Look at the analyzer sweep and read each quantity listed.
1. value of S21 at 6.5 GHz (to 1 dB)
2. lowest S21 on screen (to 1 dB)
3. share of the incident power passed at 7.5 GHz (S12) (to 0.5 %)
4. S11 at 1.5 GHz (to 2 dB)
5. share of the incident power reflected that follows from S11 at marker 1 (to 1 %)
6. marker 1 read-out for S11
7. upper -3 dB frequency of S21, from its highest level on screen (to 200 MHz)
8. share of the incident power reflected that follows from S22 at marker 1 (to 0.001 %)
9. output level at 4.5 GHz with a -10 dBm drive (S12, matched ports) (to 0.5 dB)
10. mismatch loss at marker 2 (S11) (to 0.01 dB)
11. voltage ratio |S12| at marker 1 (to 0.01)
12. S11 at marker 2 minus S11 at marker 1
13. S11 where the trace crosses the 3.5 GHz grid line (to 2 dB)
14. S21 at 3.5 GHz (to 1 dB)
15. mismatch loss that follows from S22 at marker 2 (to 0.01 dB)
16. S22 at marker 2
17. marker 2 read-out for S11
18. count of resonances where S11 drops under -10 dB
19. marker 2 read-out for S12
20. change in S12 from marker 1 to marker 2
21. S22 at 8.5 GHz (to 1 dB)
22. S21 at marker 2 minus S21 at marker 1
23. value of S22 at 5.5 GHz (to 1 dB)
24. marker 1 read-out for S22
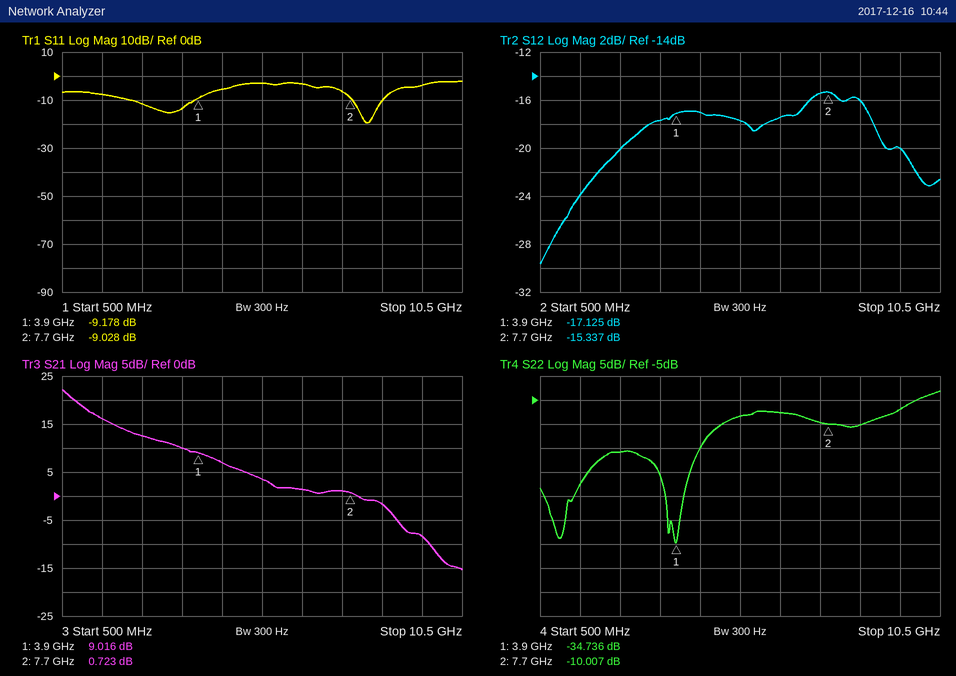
1 dB
-15 dB
3.0 %
-8 dB
12 %
-9.178 dB
1.0 GHz
0.034 %
-27.0 dBm
0.58 dB
0.14
0.150 dB
-14 dB
10 dB
0.46 dB
-10.007 dB
-9.028 dB
2
-15.337 dB
1.788 dB
-10 dB
-8.293 dB
-8 dB
-34.736 dB
